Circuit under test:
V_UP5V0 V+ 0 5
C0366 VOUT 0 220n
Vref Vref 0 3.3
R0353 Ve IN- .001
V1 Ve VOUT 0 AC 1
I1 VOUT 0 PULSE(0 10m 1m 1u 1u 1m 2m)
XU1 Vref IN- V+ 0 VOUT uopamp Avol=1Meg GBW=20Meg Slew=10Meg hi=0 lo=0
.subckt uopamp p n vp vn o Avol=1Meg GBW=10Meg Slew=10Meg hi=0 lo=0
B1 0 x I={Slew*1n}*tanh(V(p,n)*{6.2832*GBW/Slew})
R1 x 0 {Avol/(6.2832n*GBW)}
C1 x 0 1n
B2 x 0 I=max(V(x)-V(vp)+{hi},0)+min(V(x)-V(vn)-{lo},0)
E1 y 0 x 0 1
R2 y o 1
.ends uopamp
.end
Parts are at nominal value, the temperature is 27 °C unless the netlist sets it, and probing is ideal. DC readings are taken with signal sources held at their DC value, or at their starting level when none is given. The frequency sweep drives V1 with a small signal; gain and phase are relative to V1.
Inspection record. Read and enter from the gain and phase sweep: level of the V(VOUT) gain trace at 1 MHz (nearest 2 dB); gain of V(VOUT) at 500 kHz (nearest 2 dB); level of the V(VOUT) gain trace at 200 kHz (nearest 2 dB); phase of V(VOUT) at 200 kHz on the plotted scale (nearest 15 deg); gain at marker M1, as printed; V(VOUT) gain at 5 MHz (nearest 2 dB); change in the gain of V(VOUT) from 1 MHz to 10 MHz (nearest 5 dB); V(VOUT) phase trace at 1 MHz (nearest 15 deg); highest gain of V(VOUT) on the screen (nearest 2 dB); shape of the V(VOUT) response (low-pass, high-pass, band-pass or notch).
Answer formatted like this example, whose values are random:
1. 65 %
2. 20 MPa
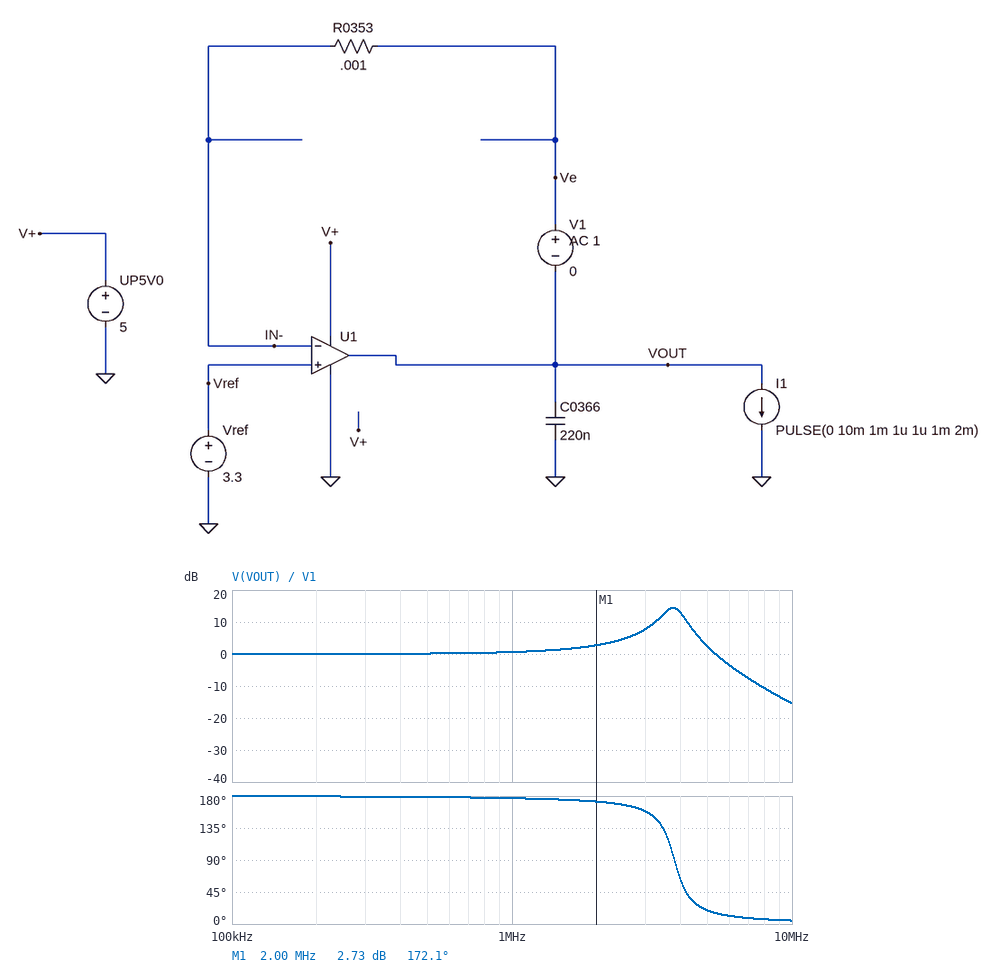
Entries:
1. 0 dB
2. 0 dB
3. 0 dB
4. 180 deg
5. 2.73 dB
6. 2 dB
7. -15 dB
8. 180 deg
9. 14 dB
10. low-pass
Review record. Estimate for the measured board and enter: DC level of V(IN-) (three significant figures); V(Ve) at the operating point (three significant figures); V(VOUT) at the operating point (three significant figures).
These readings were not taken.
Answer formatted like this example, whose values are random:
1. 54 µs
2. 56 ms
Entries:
1. 3.30 V
2. 3.30 V
3. 3.30 V
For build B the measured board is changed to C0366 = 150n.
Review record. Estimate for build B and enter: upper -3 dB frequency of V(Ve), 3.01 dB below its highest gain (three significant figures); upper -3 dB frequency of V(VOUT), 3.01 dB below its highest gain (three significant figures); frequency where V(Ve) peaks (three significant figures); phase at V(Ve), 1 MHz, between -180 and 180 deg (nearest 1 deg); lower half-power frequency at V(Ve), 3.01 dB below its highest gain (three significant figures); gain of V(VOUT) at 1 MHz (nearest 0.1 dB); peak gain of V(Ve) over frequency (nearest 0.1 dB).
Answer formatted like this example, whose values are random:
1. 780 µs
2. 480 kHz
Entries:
1. 5.33 MHz
2. 5.05 MHz
3. 4.67 MHz
4. 130 deg
5. 4.20 MHz
6. 0.4 dB
7. 13.0 dB
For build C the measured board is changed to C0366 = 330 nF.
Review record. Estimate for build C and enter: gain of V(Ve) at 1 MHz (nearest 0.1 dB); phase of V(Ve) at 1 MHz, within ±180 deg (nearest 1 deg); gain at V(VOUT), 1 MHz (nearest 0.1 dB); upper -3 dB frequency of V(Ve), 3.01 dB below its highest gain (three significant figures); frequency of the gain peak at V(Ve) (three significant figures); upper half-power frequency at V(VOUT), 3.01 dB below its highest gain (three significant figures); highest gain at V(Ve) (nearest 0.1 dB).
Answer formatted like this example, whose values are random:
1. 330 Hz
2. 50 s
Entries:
1. -17.8 dB
2. 151 deg
3. 0.9 dB
4. 3.40 MHz
5. 3.12 MHz
6. 3.32 MHz
7. 16.3 dB
